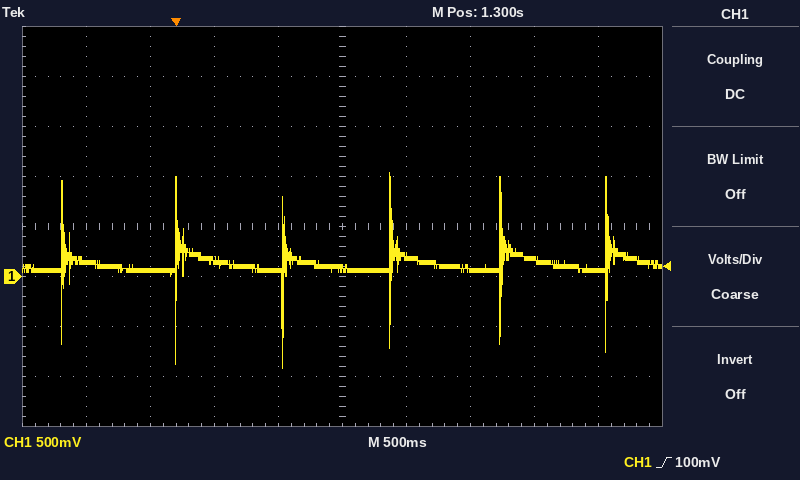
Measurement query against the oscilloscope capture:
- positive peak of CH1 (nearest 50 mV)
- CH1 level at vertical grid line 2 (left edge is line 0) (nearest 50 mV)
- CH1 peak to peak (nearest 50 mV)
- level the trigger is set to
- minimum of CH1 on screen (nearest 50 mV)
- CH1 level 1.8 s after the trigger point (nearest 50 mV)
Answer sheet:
1.05 V
50 mV
1.95 V
100 mV
-900 mV
200 mV
